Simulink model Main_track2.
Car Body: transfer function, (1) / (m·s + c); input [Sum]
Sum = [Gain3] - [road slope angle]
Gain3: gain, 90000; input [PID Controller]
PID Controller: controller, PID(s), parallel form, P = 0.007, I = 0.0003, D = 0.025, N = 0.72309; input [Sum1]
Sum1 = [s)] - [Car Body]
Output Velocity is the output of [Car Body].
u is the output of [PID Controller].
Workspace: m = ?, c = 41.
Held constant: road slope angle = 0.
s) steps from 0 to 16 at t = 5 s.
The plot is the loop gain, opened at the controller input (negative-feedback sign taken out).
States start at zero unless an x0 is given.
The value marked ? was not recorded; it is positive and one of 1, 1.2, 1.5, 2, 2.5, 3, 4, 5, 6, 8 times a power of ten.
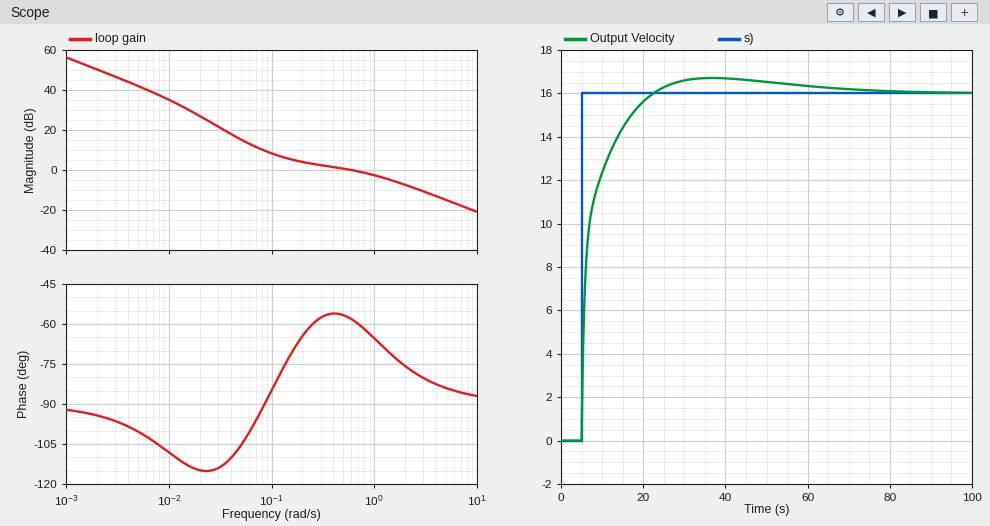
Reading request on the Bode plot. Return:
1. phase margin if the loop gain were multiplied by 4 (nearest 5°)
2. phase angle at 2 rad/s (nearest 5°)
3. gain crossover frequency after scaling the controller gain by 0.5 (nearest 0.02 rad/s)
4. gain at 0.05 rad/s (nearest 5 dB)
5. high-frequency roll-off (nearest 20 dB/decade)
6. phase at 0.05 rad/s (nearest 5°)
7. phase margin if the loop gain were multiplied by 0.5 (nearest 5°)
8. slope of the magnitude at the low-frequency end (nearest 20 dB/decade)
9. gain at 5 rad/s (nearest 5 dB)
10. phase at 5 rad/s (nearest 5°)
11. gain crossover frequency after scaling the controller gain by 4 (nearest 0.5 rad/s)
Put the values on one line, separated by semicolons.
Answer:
100°; -75°; 0.14 rad/s; 15 dB; -20 dB/decade; -105°; 105°; -20 dB/decade; -15 dB; -85°; 3.5 rad/s
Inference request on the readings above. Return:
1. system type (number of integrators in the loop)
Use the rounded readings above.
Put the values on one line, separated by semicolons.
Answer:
1
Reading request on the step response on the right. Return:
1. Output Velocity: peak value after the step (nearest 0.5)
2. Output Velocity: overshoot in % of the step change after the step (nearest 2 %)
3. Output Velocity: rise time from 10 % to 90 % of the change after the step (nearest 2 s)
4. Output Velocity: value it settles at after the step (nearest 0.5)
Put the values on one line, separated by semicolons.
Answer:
16.5; 4 %; 10 s; 16.0
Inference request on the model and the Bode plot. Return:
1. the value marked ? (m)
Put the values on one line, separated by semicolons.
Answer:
2500
